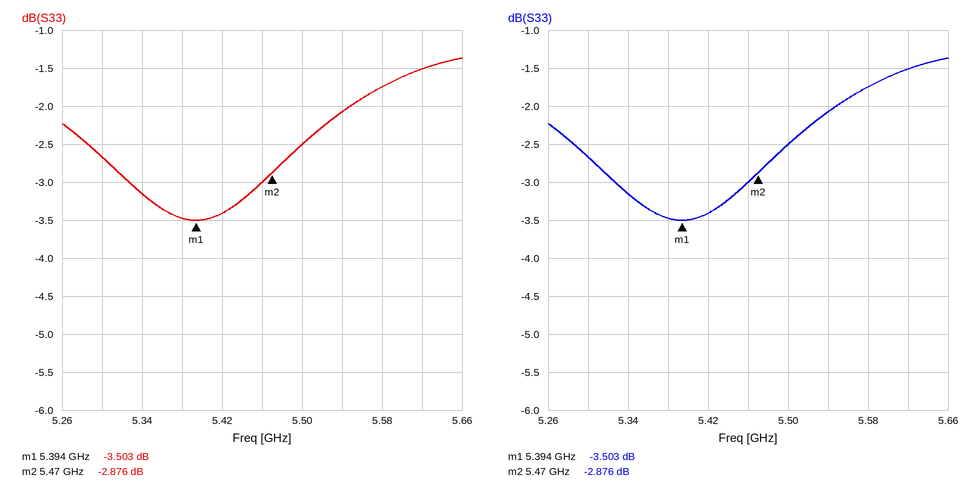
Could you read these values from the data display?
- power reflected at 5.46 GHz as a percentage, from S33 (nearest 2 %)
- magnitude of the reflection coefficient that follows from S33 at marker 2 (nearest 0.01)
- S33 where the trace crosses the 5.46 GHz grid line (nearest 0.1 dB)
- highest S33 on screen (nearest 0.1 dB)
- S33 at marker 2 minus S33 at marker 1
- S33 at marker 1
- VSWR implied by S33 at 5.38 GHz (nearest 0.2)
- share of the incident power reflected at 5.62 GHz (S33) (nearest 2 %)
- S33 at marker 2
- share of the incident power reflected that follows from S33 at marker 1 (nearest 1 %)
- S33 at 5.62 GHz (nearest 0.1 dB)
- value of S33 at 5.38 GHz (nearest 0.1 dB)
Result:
50 %
0.72
-3.0 dB
-1.4 dB
0.627 dB
-3.503 dB
5.0
70 %
-2.876 dB
45 %
-1.5 dB
-3.5 dB
